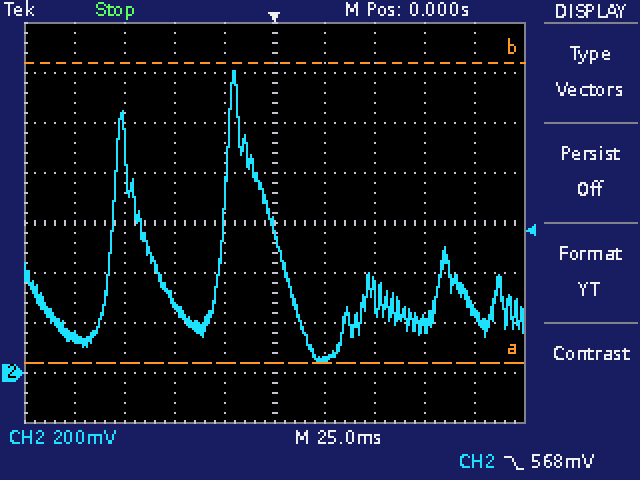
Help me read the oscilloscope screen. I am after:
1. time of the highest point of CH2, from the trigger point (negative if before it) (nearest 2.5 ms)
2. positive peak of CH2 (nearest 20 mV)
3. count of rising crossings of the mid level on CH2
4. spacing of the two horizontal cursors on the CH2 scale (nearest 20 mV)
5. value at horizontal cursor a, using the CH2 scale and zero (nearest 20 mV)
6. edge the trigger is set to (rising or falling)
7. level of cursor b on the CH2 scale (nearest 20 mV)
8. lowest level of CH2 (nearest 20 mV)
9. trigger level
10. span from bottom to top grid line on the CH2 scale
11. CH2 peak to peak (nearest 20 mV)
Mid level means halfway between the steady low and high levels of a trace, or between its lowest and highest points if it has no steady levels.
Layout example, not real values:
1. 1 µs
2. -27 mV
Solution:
1. -20.0 ms
2. 1.20 V
3. 2
4. 1.20 V
5. 40 mV
6. falling
7. 1.24 V
8. 40 mV
9. 568 mV
10. 1.6 V
11. 1.16 V
